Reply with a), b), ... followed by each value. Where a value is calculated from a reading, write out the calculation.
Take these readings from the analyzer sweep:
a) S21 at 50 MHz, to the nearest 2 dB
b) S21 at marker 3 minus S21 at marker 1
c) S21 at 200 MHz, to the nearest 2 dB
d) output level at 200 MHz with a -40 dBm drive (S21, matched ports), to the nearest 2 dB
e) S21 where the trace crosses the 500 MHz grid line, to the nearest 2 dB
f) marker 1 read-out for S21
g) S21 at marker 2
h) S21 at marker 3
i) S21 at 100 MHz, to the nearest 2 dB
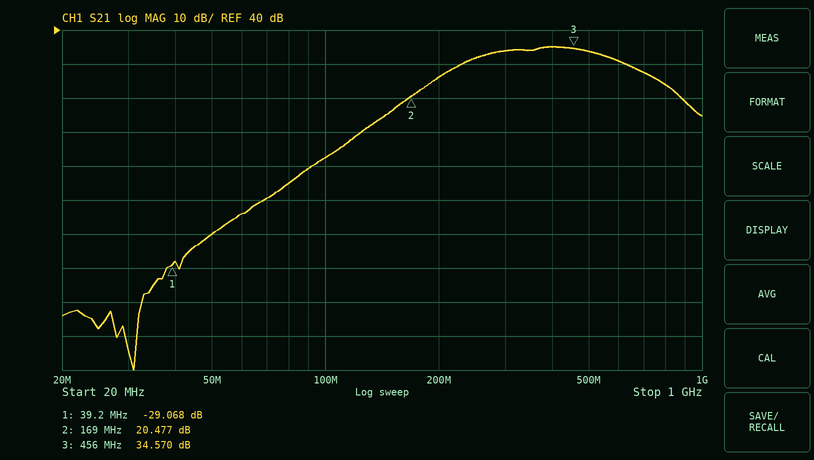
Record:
a) -20 dB
b) 34.57 − (-29.068) = 63.638 dB
c) 26 dB
d) -40 dBm + (26 dB) = -14 dBm
e) 34 dB
f) -29.068 dB
g) 20.477 dB
h) 34.570 dB
i) 2 dB
